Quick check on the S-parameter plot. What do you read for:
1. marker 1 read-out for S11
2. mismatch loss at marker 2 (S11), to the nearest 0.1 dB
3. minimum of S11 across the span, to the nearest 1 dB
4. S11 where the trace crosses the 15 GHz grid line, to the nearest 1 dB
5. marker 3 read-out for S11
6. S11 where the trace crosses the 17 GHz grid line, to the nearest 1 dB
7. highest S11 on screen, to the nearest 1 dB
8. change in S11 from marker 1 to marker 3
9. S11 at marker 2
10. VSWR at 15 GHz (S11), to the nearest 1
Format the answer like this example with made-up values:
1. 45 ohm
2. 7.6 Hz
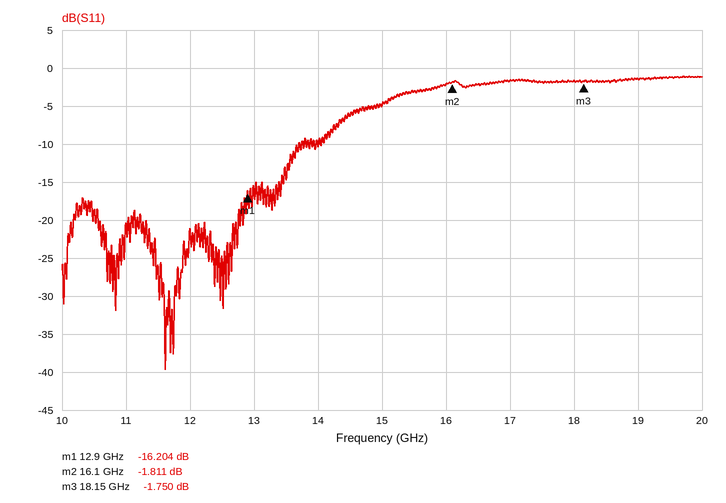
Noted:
1. -16.204 dB
2. 4.7 dB
3. -40 dB
4. -5 dB
5. -1.750 dB
6. -2 dB
7. -1 dB
8. 14.454 dB
9. -1.811 dB
10. 4
